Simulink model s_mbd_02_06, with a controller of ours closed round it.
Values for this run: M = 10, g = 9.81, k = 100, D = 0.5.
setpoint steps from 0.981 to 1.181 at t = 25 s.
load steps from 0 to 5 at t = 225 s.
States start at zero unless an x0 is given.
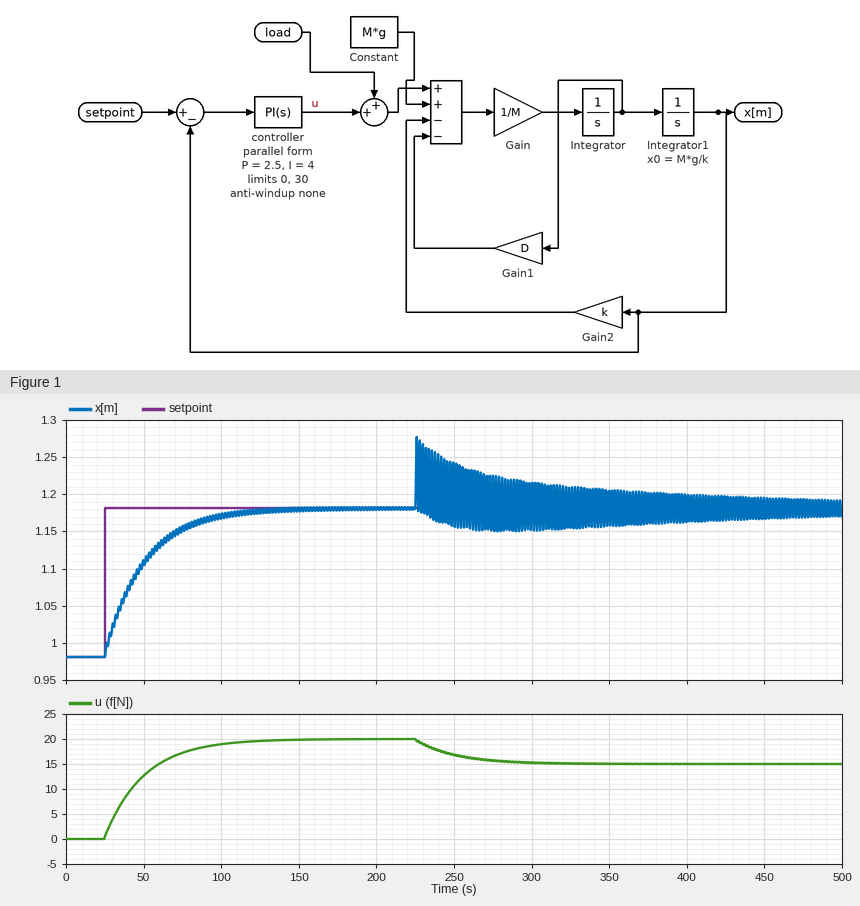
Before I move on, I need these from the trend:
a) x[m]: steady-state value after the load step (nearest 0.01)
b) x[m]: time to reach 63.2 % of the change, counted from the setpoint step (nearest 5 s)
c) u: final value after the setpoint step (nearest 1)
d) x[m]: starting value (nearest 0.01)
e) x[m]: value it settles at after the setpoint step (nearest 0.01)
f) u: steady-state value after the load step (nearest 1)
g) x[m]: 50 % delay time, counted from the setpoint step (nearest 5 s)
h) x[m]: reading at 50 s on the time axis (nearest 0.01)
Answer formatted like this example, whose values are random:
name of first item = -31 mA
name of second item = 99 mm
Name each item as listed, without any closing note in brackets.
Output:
x[m]: steady-state value after the load step = 1.18
x[m]: time to reach 63.2 % of the change, counted from the setpoint step = 25 s
u: final value after the setpoint step = 20
x[m]: starting value = 0.98
x[m]: value it settles at after the setpoint step = 1.18
u: steady-state value after the load step = 15
x[m]: 50 % delay time, counted from the setpoint step = 15 s
x[m]: reading at 50 s on the time axis = 1.11
